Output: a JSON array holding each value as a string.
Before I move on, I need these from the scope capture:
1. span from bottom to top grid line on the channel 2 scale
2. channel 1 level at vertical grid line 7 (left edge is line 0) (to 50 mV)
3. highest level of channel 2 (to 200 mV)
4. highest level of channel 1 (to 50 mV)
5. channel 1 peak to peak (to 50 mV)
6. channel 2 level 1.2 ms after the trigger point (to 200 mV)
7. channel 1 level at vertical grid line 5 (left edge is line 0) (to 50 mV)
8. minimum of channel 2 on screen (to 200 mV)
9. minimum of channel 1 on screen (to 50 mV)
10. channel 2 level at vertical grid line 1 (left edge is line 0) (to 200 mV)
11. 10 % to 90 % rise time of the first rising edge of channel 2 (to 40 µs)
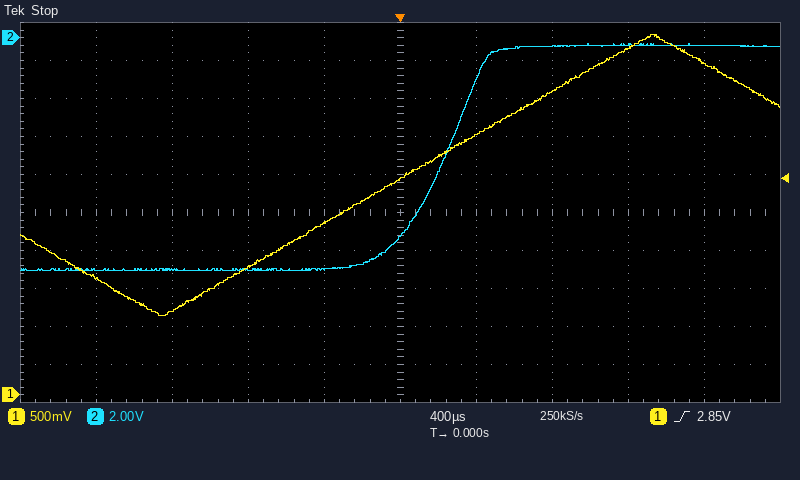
["20 V", "4.00 V", "-400 mV", "4.75 V", "3.70 V", "-400 mV", "2.85 V", "-12.2 V", "1.05 V", "-12.2 V", "480 µs"]
